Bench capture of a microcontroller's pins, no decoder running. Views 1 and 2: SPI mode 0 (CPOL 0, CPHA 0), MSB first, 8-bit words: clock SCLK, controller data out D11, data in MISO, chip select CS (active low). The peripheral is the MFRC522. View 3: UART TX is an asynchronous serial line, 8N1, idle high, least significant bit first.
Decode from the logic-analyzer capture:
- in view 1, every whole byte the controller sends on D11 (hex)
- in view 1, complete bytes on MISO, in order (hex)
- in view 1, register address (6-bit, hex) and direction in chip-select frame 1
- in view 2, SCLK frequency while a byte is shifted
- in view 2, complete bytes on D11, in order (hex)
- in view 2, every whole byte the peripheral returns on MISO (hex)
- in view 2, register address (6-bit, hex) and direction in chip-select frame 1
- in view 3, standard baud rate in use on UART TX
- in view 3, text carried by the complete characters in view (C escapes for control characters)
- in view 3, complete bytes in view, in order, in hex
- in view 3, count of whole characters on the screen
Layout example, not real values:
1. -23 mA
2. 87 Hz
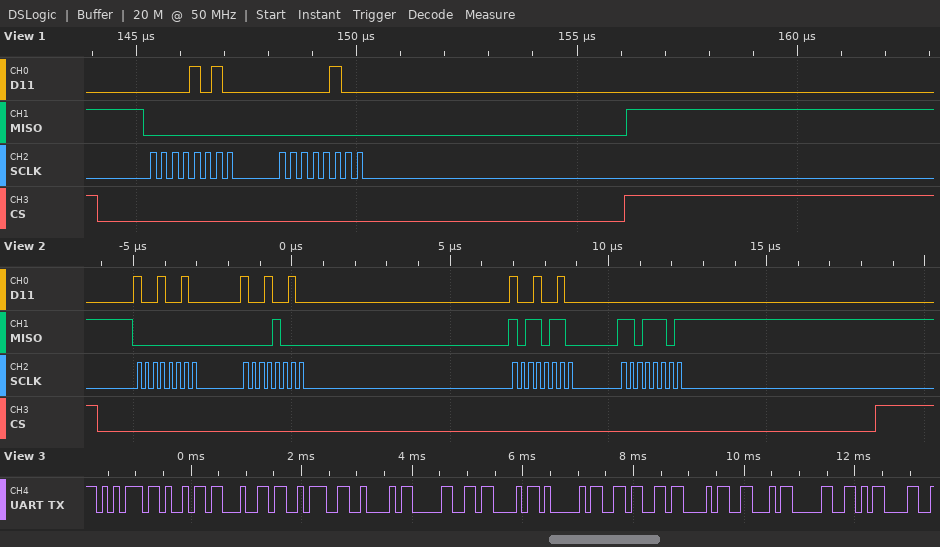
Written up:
1. 0x0A 0x04
2. 0x00 0x00
3. 0x05 write
4. 4 MHz
5. 92 92 92 00
6. 00 08 B6 DD
7. 0x09 read
8. 9600 baud
9. "uid:B0CA6CF0\r"
10. 75 69 64 3A 42 30 43 41 36 43 46 30 0D
11. 13
